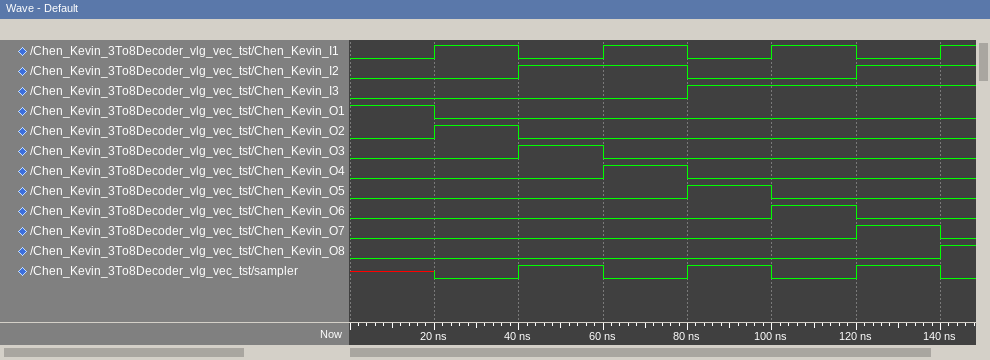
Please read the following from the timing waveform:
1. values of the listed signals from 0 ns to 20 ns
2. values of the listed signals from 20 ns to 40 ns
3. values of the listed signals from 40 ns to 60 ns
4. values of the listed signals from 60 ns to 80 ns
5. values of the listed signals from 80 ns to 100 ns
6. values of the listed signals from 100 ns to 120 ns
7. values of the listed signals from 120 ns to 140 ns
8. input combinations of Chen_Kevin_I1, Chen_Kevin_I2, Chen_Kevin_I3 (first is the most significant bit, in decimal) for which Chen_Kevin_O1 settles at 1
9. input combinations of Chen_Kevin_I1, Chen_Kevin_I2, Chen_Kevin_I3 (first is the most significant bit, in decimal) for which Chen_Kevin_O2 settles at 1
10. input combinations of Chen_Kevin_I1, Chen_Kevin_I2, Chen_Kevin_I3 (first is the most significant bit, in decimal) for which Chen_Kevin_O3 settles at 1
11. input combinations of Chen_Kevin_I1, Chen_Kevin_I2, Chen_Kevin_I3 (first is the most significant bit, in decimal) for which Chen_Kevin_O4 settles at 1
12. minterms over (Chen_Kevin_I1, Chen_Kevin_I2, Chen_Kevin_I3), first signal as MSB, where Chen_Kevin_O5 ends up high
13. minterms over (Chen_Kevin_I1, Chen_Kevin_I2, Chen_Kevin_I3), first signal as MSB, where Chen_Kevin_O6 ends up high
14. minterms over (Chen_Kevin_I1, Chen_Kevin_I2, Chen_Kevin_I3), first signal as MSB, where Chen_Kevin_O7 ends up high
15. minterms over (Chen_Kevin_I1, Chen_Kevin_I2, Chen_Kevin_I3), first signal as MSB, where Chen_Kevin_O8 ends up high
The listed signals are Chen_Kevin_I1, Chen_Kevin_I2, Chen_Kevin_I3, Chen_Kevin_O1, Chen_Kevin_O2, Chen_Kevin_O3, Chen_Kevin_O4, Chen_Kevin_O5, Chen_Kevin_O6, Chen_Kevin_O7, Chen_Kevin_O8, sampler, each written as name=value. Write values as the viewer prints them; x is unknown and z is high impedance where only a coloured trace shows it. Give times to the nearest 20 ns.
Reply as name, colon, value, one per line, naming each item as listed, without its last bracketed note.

values of the listed signals from 0 ns to 20 ns: Chen_Kevin_I1=0, Chen_Kevin_I2=0, Chen_Kevin_I3=0, Chen_Kevin_O1=1, Chen_Kevin_O2=0, Chen_Kevin_O3=0, Chen_Kevin_O4=0, Chen_Kevin_O5=0, Chen_Kevin_O6=0, Chen_Kevin_O7=0, Chen_Kevin_O8=0, sampler=x
values of the listed signals from 20 ns to 40 ns: Chen_Kevin_I1=1, Chen_Kevin_I2=0, Chen_Kevin_I3=0, Chen_Kevin_O1=0, Chen_Kevin_O2=1, Chen_Kevin_O3=0, Chen_Kevin_O4=0, Chen_Kevin_O5=0, Chen_Kevin_O6=0, Chen_Kevin_O7=0, Chen_Kevin_O8=0, sampler=0
values of the listed signals from 40 ns to 60 ns: Chen_Kevin_I1=0, Chen_Kevin_I2=1, Chen_Kevin_I3=0, Chen_Kevin_O1=0, Chen_Kevin_O2=0, Chen_Kevin_O3=1, Chen_Kevin_O4=0, Chen_Kevin_O5=0, Chen_Kevin_O6=0, Chen_Kevin_O7=0, Chen_Kevin_O8=0, sampler=1
values of the listed signals from 60 ns to 80 ns: Chen_Kevin_I1=1, Chen_Kevin_I2=1, Chen_Kevin_I3=0, Chen_Kevin_O1=0, Chen_Kevin_O2=0, Chen_Kevin_O3=0, Chen_Kevin_O4=1, Chen_Kevin_O5=0, Chen_Kevin_O6=0, Chen_Kevin_O7=0, Chen_Kevin_O8=0, sampler=0
values of the listed signals from 80 ns to 100 ns: Chen_Kevin_I1=0, Chen_Kevin_I2=0, Chen_Kevin_I3=1, Chen_Kevin_O1=0, Chen_Kevin_O2=0, Chen_Kevin_O3=0, Chen_Kevin_O4=0, Chen_Kevin_O5=1, Chen_Kevin_O6=0, Chen_Kevin_O7=0, Chen_Kevin_O8=0, sampler=1
values of the listed signals from 100 ns to 120 ns: Chen_Kevin_I1=1, Chen_Kevin_I2=0, Chen_Kevin_I3=1, Chen_Kevin_O1=0, Chen_Kevin_O2=0, Chen_Kevin_O3=0, Chen_Kevin_O4=0, Chen_Kevin_O5=0, Chen_Kevin_O6=1, Chen_Kevin_O7=0, Chen_Kevin_O8=0, sampler=0
values of the listed signals from 120 ns to 140 ns: Chen_Kevin_I1=0, Chen_Kevin_I2=1, Chen_Kevin_I3=1, Chen_Kevin_O1=0, Chen_Kevin_O2=0, Chen_Kevin_O3=0, Chen_Kevin_O4=0, Chen_Kevin_O5=0, Chen_Kevin_O6=0, Chen_Kevin_O7=1, Chen_Kevin_O8=0, sampler=1
input combinations of Chen_Kevin_I1, Chen_Kevin_I2, Chen_Kevin_I3 (first is the most significant bit, in decimal) for which Chen_Kevin_O1 settles at 1: 0
input combinations of Chen_Kevin_I1, Chen_Kevin_I2, Chen_Kevin_I3 (first is the most significant bit, in decimal) for which Chen_Kevin_O2 settles at 1: 4
input combinations of Chen_Kevin_I1, Chen_Kevin_I2, Chen_Kevin_I3 (first is the most significant bit, in decimal) for which Chen_Kevin_O3 settles at 1: 2
input combinations of Chen_Kevin_I1, Chen_Kevin_I2, Chen_Kevin_I3 (first is the most significant bit, in decimal) for which Chen_Kevin_O4 settles at 1: 6
minterms over (Chen_Kevin_I1, Chen_Kevin_I2, Chen_Kevin_I3), first signal as MSB, where Chen_Kevin_O5 ends up high: 1
minterms over (Chen_Kevin_I1, Chen_Kevin_I2, Chen_Kevin_I3), first signal as MSB, where Chen_Kevin_O6 ends up high: 5
minterms over (Chen_Kevin_I1, Chen_Kevin_I2, Chen_Kevin_I3), first signal as MSB, where Chen_Kevin_O7 ends up high: 3
minterms over (Chen_Kevin_I1, Chen_Kevin_I2, Chen_Kevin_I3), first signal as MSB, where Chen_Kevin_O8 ends up high: 7
